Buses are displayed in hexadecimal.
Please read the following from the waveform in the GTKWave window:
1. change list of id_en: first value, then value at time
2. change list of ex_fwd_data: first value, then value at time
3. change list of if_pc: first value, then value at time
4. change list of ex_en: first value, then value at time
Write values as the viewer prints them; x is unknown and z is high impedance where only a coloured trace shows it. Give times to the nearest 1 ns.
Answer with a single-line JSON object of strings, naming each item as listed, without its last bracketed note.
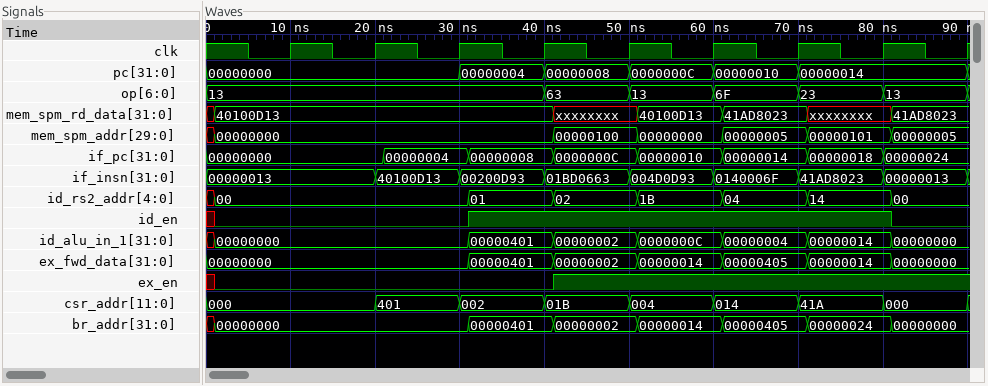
{"change list of id_en: first value, then value at time": "x, 0 at 1 ns, 1 at 31 ns, 0 at 81 ns", "change list of ex_fwd_data: first value, then value at time": "00000000, 00000401 at 31 ns, 00000002 at 41 ns, 00000014 at 51 ns, 00000405 at 61 ns, 00000014 at 71 ns, 00000000 at 81 ns", "change list of if_pc: first value, then value at time": "00000000, 00000004 at 21 ns, 00000008 at 31 ns, 0000000C at 41 ns, 00000010 at 51 ns, 00000014 at 61 ns, 00000018 at 71 ns, 00000024 at 80 ns", "change list of ex_en: first value, then value at time": "x, 0 at 1 ns, 1 at 41 ns"}
